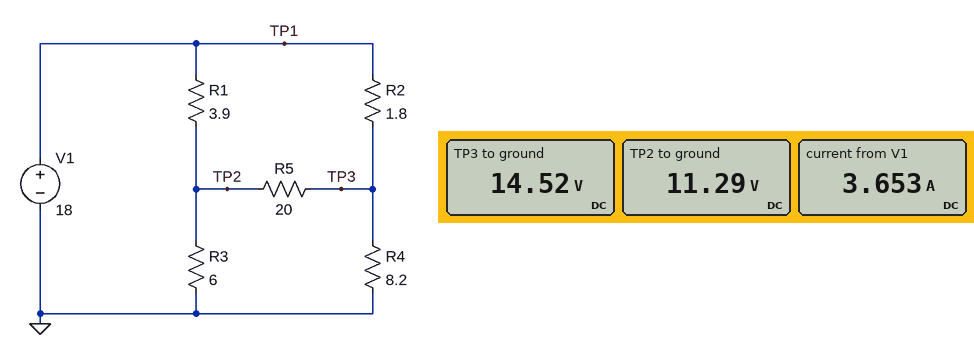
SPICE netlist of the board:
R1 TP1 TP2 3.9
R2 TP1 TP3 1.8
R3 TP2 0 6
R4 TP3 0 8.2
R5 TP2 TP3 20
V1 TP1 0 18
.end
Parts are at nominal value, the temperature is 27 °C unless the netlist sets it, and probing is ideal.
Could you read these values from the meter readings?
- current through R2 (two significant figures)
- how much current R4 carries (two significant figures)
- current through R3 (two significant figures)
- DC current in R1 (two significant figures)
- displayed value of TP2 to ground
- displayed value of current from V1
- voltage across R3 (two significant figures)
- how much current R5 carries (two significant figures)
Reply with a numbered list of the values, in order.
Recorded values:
1. 1.9 A
2. 1.8 A
3. 1.9 A
4. 1.7 A
5. 11.29 V
6. 3.653 A
7. 11 V
8. 160 mA
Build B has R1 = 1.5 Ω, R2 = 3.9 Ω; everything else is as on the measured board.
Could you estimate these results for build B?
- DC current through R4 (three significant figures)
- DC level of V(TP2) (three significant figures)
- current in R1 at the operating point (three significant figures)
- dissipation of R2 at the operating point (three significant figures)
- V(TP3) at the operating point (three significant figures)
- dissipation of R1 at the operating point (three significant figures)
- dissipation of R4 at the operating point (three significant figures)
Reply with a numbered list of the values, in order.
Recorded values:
1. 1.52 A
2. 14.3 V
3. 2.47 A
4. 7.92 W
5. 12.4 V
6. 9.18 W
7. 18.9 W
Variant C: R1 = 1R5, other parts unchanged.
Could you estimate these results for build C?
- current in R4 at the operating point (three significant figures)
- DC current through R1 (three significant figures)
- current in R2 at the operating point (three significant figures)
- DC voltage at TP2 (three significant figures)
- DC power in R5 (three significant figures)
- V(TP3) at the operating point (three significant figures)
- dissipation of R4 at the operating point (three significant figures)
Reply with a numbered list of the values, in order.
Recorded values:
1. 1.80 A
2. 2.39 A
3. 1.81 A
4. 14.4 V
5. 5.04 mW
6. 14.7 V
7. 26.5 W
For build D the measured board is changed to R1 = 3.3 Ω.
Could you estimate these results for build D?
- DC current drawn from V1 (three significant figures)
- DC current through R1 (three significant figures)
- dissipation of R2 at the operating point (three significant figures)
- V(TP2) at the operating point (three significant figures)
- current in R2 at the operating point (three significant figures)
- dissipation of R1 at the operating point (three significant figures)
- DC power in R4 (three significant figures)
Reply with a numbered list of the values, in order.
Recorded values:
1. 3.76 A
2. 1.85 A
3. 6.56 W
4. 11.9 V
5. 1.91 A
6. 11.3 W
7. 25.9 W
